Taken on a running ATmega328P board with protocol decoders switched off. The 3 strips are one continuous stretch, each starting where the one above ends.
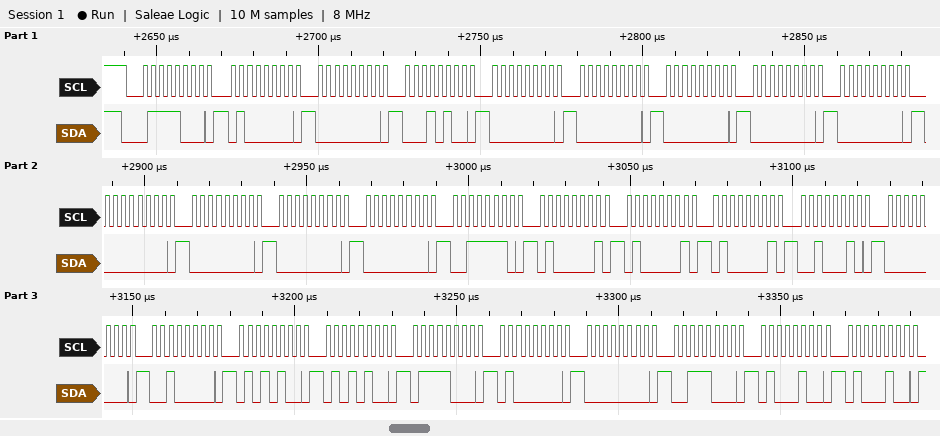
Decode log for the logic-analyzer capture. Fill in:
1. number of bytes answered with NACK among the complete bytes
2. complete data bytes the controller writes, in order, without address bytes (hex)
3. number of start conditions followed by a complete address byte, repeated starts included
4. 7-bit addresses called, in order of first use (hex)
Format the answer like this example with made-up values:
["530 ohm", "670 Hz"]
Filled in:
["0", "40 00 14 00 00 00 00 00 00 00 00 00 3E 41 41 41 22 00 20 54 54 78 40 00 38 44 44", "1", "0x3C"]
